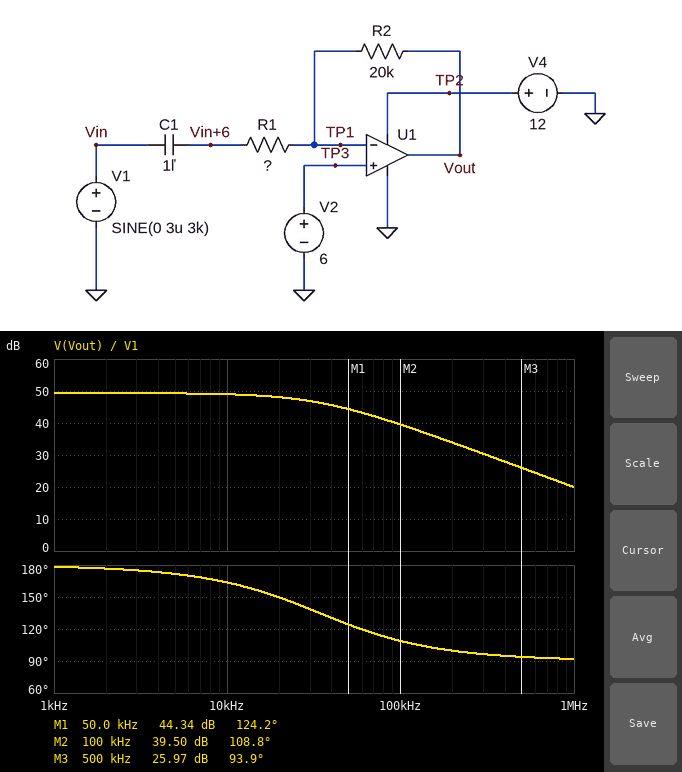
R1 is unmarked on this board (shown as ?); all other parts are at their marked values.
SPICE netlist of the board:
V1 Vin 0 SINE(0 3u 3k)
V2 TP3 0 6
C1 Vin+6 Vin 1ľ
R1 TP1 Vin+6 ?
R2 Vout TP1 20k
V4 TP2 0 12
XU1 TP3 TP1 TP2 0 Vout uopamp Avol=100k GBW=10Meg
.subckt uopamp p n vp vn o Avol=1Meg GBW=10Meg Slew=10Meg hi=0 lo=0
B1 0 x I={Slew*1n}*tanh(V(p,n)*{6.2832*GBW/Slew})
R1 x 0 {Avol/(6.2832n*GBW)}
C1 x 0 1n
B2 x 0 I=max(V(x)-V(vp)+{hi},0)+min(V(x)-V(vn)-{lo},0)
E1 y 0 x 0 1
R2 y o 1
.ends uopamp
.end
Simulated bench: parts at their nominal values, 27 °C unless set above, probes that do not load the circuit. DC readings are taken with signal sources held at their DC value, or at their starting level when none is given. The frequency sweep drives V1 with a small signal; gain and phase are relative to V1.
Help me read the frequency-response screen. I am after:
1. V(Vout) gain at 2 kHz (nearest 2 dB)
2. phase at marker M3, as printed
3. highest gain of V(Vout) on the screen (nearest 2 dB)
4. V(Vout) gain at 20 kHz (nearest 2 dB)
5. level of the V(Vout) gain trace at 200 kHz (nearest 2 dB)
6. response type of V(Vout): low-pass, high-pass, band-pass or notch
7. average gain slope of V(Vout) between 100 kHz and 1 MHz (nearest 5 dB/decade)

50 dB
93.9 deg
50 dB
48 dB
34 dB
low-pass
-20 dB/decade
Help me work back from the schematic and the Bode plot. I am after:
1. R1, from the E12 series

68 Ω
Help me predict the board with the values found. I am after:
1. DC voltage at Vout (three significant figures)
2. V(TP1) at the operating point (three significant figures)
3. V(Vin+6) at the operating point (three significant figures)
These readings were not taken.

6.00 V
6.00 V
6.00 V
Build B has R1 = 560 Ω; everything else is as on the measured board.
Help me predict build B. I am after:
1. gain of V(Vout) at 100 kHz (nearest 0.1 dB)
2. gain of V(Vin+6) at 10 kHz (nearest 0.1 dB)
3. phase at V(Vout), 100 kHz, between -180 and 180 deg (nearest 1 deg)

30.5 dB
0 dB
160 deg
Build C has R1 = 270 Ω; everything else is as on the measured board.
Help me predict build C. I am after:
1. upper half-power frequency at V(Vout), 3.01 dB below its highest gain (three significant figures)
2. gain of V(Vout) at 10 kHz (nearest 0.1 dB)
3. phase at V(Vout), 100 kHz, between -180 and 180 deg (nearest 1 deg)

133 kHz
37.4 dB
143 deg
